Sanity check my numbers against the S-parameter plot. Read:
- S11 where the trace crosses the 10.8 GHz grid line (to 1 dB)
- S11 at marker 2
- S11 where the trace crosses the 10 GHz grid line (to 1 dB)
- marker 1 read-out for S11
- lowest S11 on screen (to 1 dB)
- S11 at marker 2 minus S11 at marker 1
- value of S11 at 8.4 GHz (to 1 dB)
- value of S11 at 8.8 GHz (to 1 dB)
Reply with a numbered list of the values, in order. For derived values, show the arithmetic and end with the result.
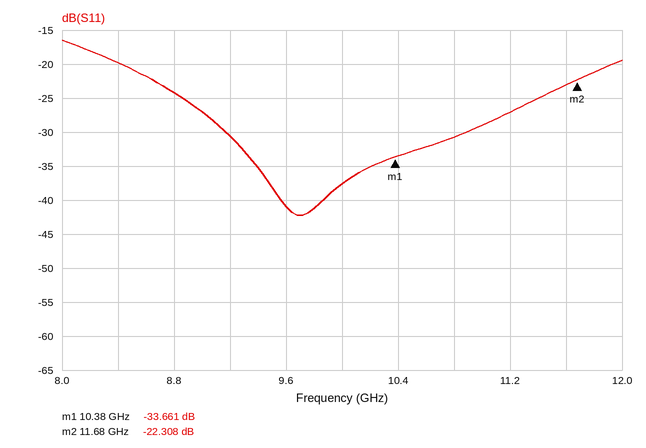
1. -31 dB
2. -22.308 dB
3. -38 dB
4. -33.661 dB
5. -42 dB
6. -22.308 − (-33.661) = 11.353 dB
7. -20 dB
8. -24 dB
